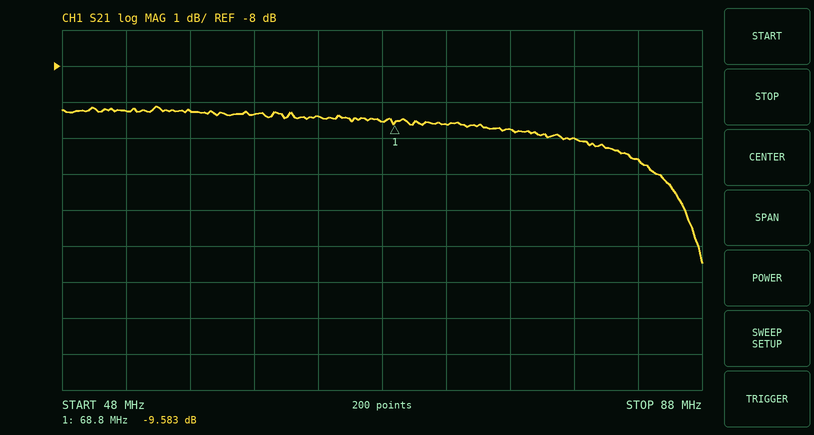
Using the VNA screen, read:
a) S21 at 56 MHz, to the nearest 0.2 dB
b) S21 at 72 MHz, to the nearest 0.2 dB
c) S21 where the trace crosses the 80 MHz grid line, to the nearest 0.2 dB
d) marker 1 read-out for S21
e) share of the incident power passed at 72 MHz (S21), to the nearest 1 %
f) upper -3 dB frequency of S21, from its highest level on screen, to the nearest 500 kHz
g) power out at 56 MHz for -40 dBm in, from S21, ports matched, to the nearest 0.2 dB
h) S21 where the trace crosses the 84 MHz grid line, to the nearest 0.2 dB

-9.2 dB
-9.6 dB
-10.0 dB
-9.583 dB
11 %
87.0 MHz
-49.2 dBm
-10.6 dB
